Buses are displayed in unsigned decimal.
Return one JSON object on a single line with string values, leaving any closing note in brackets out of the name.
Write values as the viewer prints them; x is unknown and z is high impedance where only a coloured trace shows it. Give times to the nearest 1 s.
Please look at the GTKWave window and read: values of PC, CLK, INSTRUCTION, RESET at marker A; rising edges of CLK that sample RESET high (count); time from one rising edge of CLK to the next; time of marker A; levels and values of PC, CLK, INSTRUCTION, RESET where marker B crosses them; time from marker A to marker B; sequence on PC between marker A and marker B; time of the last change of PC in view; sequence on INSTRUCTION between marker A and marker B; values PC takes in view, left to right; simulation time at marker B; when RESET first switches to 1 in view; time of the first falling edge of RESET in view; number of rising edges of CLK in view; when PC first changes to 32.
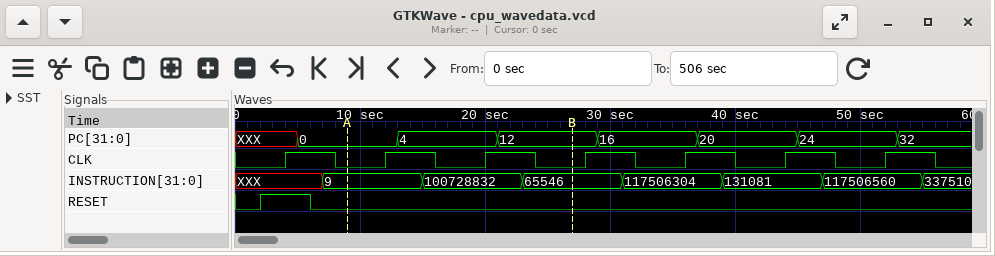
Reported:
{"values of PC, CLK, INSTRUCTION, RESET at marker A": "PC=0, CLK=0, INSTRUCTION=9, RESET=0", "rising edges of CLK that sample RESET high": "1", "time from one rising edge of CLK to the next": "8 s", "time of marker A": "9 s", "levels and values of PC, CLK, INSTRUCTION, RESET where marker B crosses them": "PC=12, CLK=0, INSTRUCTION=65546, RESET=0", "time from marker A to marker B": "18 s", "sequence on PC between marker A and marker B": "0, 4, 12", "time of the last change of PC in view": "53 s", "sequence on INSTRUCTION between marker A and marker B": "9, 100728832, 65546", "values PC takes in view, left to right": "XXX, 0, 4, 12, 16, 20, 24, 32", "simulation time at marker B": "27 s", "when RESET first switches to 1 in view": "2 s", "time of the first falling edge of RESET in view": "6 s", "number of rising edges of CLK in view": "7", "when PC first changes to 32": "53 s"}
